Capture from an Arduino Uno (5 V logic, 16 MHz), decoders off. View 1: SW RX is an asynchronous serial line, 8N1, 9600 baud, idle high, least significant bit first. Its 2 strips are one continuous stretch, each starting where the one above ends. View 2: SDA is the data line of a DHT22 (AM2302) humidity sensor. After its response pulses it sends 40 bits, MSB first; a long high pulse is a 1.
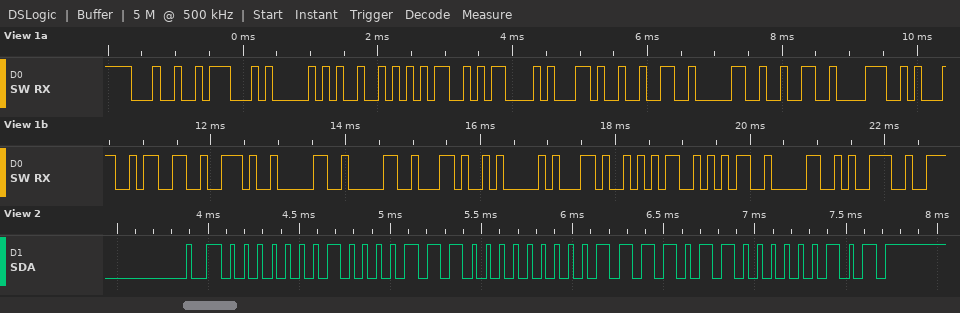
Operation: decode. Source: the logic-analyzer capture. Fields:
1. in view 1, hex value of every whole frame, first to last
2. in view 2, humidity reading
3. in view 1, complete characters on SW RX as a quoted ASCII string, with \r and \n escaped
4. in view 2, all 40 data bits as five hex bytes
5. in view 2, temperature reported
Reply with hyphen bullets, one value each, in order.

- 24 47 50 52 4D 43 2C 32 30 32 38 31 33 2E 30 30 2C 41 2C 35 35 30 39
- 27.0 %
- "$GPRMC,202813.00,A,5509"
- 01 0E 00 F6 05
- 24.6 °C
